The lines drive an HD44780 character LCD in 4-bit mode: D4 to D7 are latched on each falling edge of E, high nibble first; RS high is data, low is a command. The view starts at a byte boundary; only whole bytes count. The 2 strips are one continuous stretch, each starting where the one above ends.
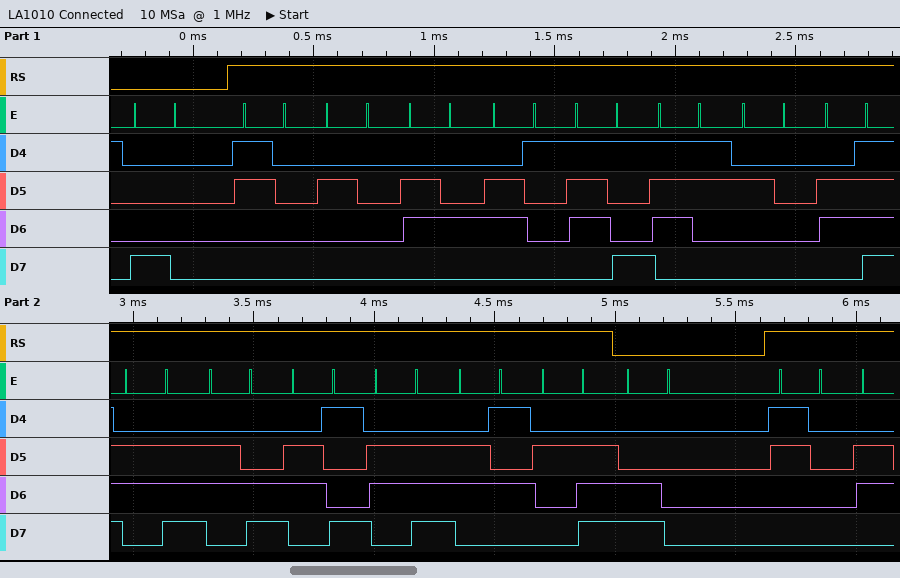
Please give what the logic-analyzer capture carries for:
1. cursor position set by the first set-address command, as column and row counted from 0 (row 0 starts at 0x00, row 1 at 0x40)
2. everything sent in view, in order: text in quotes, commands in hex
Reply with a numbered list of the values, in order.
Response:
1. column 0, row 0
2. 0x80 "0 days online." 0xC0 "0"
